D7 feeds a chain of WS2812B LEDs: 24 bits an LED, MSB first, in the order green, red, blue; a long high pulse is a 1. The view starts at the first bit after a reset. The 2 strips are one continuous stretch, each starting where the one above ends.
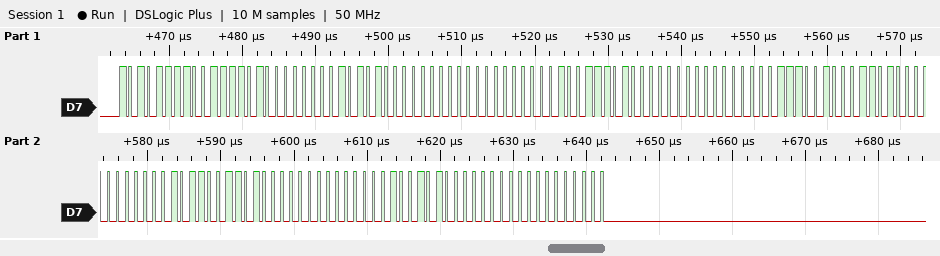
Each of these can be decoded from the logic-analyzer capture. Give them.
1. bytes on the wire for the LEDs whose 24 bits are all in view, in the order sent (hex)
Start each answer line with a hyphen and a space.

- AF 3D 00 A8 00 00 9D 00 00 E4 68 00 B3 40 00 94 00 00
